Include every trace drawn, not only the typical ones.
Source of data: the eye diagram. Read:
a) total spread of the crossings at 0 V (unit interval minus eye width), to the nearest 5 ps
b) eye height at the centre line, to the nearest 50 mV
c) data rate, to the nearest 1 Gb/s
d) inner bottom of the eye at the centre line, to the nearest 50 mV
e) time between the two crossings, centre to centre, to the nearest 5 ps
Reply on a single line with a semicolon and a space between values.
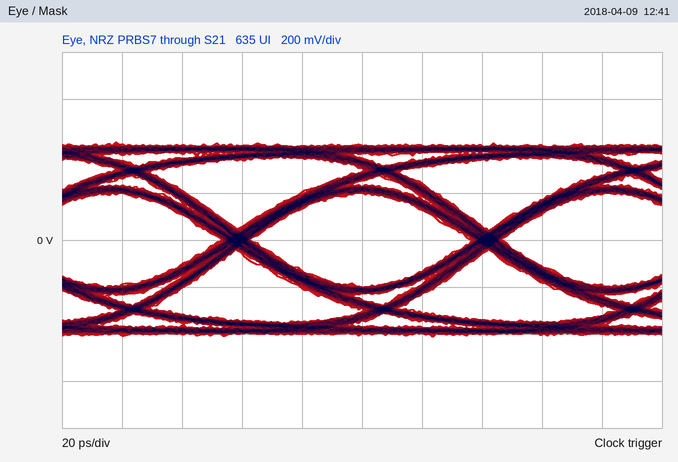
10 ps; 400 mV; 12 Gb/s; -200 mV; 85 ps
